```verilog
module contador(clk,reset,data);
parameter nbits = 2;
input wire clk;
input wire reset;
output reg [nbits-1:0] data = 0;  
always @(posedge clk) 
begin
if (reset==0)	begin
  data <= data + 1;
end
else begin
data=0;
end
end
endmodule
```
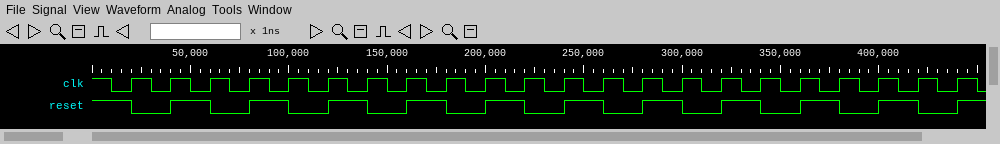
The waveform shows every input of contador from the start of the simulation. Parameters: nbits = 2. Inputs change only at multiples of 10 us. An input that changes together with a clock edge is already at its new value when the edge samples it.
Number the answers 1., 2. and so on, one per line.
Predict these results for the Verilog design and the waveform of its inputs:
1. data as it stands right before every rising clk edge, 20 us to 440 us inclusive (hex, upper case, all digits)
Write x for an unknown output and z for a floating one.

1. 0, 1, 0, 1, 0, 1, 0, 1, 0, 1, 0, 1, 0, 1, 0, 1, 0, 1, 0, 1, 0, 1
